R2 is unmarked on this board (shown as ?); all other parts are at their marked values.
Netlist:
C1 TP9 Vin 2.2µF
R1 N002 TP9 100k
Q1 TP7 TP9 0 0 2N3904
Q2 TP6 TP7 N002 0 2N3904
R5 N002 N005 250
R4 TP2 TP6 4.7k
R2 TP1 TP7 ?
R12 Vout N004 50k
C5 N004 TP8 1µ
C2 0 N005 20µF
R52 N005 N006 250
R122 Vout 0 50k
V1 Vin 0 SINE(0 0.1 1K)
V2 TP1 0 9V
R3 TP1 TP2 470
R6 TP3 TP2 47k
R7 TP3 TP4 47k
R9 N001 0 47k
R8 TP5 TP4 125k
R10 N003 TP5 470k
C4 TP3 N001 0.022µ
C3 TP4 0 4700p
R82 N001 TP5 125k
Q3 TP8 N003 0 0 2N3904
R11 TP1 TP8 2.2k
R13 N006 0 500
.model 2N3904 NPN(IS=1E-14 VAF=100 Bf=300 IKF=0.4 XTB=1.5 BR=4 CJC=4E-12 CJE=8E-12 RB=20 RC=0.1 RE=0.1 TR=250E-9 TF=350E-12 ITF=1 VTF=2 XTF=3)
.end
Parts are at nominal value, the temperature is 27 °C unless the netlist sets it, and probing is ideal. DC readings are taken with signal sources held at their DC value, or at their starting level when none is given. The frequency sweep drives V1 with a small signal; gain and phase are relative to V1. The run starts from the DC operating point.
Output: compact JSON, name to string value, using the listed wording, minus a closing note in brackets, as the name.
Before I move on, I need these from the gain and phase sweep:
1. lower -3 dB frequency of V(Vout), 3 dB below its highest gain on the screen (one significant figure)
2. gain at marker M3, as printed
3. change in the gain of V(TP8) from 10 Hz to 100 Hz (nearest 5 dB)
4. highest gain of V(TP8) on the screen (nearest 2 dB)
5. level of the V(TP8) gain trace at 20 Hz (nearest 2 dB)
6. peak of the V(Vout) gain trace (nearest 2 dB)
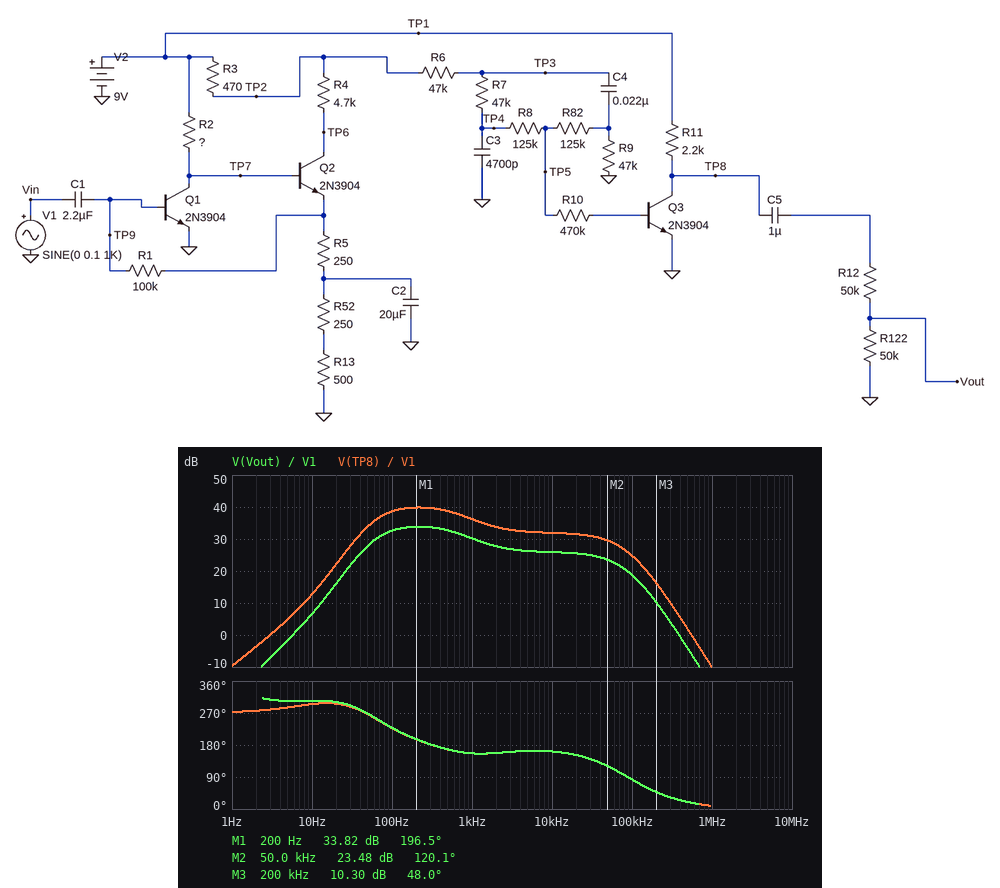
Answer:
{"lower -3 dB frequency of V(Vout), 3 dB below its highest gain on the screen": "70 Hz", "gain at marker M3, as printed": "10.30 dB", "change in the gain of V(TP8) from 10 Hz to 100 Hz": "25 dB", "highest gain of V(TP8) on the screen": "40 dB", "level of the V(TP8) gain trace at 20 Hz": "22 dB", "peak of the V(Vout) gain trace": "34 dB"}
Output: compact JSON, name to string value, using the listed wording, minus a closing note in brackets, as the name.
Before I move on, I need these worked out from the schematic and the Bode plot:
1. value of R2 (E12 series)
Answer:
{"value of R2": "100 kΩ"}
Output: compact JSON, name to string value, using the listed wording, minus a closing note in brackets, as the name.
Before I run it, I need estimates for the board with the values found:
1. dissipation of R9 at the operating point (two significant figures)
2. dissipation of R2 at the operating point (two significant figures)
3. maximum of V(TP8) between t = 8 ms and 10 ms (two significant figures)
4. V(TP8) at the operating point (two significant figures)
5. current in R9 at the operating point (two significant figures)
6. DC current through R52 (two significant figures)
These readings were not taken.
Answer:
{"dissipation of R9 at the operating point": "17 µW", "dissipation of R2 at the operating point": "600 µW", "maximum of V(TP8) between t = 8 ms and 10 ms": "5.4 V", "V(TP8) at the operating point": "5.2 V", "current in R9 at the operating point": "19 µA", "DC current through R52": "610 µA"}
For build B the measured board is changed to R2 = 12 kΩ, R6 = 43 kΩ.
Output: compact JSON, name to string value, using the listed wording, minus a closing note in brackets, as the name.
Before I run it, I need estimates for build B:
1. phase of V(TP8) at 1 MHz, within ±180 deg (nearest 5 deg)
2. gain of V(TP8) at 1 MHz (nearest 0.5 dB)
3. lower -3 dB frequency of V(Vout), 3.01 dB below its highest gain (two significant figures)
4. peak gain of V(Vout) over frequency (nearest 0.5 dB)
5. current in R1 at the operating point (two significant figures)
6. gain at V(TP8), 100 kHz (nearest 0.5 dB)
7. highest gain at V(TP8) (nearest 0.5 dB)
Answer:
{"phase of V(TP8) at 1 MHz, within ±180 deg": "20 deg", "gain of V(TP8) at 1 MHz": "7.5 dB", "lower -3 dB frequency of V(Vout), 3.01 dB below its highest gain": "120 Hz", "peak gain of V(Vout) over frequency": "38.5 dB", "current in R1 at the operating point": "2.1 µA", "gain at V(TP8), 100 kHz": "34.5 dB", "highest gain at V(TP8)": "44.5 dB"}
